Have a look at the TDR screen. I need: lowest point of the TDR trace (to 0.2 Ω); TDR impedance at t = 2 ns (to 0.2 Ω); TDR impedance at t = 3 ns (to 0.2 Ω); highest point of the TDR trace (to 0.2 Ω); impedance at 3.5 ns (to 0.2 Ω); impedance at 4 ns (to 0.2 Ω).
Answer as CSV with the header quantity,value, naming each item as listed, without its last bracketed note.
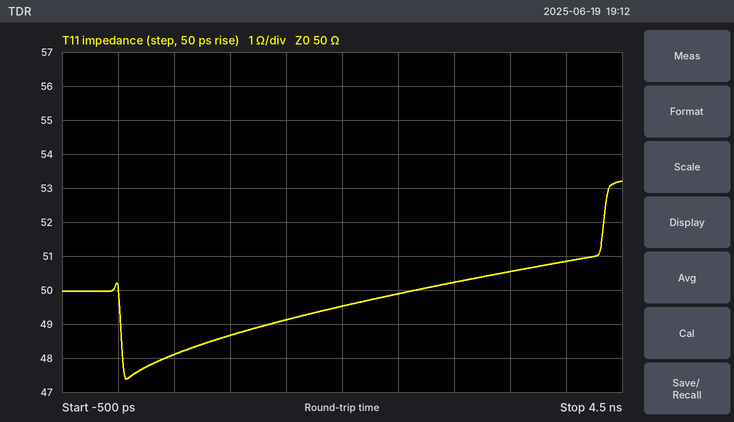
quantity,value
lowest point of the TDR trace,47.4 Ω
TDR impedance at t = 2 ns,49.6 Ω
TDR impedance at t = 3 ns,50.2 Ω
highest point of the TDR trace,53.2 Ω
impedance at 3.5 ns,50.6 Ω
impedance at 4 ns,50.8 Ω
